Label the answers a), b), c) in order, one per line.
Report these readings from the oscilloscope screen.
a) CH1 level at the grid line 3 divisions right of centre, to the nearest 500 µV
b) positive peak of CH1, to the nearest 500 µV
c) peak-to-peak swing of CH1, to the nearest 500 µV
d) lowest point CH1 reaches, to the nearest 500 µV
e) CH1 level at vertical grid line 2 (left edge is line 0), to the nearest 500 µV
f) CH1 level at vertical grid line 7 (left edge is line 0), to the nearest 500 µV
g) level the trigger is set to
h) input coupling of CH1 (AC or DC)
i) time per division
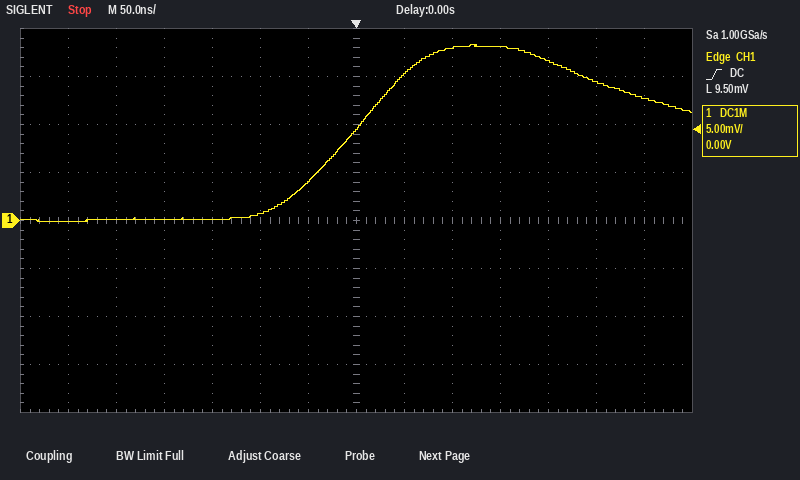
a) 18.0 mV
b) 18.5 mV
c) 18.5 mV
d) 0.0 mV
e) 0.0 mV
f) 9.5 mV
g) 9.50 mV
h) DC
i) 50 ns
